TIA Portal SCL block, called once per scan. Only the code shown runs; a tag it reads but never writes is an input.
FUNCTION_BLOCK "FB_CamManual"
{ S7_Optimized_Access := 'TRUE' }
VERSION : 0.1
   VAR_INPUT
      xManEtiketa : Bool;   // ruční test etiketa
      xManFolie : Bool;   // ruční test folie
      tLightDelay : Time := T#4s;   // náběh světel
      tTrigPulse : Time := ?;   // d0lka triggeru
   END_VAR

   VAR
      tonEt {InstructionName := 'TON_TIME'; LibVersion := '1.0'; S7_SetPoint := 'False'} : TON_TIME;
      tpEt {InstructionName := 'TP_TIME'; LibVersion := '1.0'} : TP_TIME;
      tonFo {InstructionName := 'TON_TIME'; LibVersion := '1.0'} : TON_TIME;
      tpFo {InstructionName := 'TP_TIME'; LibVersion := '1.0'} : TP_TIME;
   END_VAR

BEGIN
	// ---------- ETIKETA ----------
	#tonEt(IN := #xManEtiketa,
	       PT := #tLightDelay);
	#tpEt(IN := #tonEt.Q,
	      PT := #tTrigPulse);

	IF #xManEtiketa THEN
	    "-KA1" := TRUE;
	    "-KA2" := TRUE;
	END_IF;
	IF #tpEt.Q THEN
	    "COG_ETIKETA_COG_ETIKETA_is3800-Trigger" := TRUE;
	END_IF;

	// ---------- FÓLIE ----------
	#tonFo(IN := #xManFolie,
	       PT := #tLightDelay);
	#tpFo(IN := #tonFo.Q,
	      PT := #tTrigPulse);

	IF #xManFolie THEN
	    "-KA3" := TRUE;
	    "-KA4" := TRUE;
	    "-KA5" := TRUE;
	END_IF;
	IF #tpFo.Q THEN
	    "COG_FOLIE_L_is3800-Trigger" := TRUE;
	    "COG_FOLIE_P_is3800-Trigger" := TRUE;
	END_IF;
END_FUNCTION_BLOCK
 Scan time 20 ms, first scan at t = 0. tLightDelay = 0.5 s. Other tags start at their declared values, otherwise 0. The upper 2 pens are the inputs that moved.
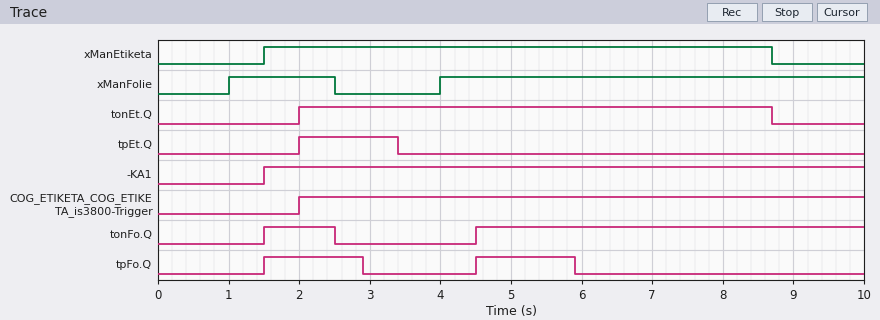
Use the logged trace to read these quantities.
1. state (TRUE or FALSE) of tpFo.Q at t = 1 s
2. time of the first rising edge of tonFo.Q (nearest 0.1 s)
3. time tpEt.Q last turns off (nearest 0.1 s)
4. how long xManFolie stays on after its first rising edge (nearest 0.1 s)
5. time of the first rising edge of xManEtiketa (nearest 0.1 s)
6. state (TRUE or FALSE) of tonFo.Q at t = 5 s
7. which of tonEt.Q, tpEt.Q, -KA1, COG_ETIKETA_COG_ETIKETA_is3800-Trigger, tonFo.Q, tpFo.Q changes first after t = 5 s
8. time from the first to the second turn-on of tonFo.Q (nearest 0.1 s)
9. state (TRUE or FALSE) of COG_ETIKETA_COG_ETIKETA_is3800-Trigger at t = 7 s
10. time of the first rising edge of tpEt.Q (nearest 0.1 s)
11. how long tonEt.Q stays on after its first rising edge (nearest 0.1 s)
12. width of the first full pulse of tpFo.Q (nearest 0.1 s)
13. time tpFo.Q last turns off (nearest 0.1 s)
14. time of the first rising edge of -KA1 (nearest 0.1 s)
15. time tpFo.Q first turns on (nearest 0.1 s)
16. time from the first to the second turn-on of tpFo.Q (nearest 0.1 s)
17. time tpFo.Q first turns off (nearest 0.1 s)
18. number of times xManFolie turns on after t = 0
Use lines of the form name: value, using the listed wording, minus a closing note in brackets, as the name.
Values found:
state (TRUE or FALSE) of tpFo.Q at t = 1 s: FALSE
time of the first rising edge of tonFo.Q: 1.5 s
time tpEt.Q last turns off: 3.4 s
how long xManFolie stays on after its first rising edge: 1.5 s
time of the first rising edge of xManEtiketa: 1.5 s
state (TRUE or FALSE) of tonFo.Q at t = 5 s: TRUE
which of tonEt.Q, tpEt.Q, -KA1, COG_ETIKETA_COG_ETIKETA_is3800-Trigger, tonFo.Q, tpFo.Q changes first after t = 5 s: tpFo.Q
time from the first to the second turn-on of tonFo.Q: 3.0 s
state (TRUE or FALSE) of COG_ETIKETA_COG_ETIKETA_is3800-Trigger at t = 7 s: TRUE
time of the first rising edge of tpEt.Q: 2.0 s
how long tonEt.Q stays on after its first rising edge: 6.7 s
width of the first full pulse of tpFo.Q: 1.4 s
time tpFo.Q last turns off: 5.9 s
time of the first rising edge of -KA1: 1.5 s
time tpFo.Q first turns on: 1.5 s
time from the first to the second turn-on of tpFo.Q: 3.0 s
time tpFo.Q first turns off: 2.9 s
number of times xManFolie turns on after t = 0: 2
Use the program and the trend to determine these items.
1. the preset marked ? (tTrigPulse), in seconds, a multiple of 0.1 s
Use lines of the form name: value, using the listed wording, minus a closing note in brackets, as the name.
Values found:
the preset marked ? (tTrigPulse), in seconds, a multiple of 0.1 s: 1.4 s
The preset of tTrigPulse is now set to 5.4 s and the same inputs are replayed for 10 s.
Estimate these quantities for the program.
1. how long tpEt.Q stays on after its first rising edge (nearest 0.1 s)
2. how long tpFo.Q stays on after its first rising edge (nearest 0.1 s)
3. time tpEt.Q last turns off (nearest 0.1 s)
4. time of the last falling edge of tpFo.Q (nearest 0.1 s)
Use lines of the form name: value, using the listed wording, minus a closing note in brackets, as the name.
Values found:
how long tpEt.Q stays on after its first rising edge: 5.4 s
how long tpFo.Q stays on after its first rising edge: 5.4 s
time tpEt.Q last turns off: 7.4 s
time of the last falling edge of tpFo.Q: 6.9 s
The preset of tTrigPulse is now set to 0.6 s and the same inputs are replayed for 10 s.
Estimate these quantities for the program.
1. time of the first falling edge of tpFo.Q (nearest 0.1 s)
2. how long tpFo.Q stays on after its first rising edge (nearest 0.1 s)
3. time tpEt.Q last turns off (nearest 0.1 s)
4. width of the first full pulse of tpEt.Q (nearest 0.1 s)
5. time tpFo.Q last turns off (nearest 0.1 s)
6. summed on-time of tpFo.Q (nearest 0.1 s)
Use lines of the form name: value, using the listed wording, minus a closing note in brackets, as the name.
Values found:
time of the first falling edge of tpFo.Q: 2.1 s
how long tpFo.Q stays on after its first rising edge: 0.6 s
time tpEt.Q last turns off: 2.6 s
width of the first full pulse of tpEt.Q: 0.6 s
time tpFo.Q last turns off: 5.1 s
summed on-time of tpFo.Q: 1.2 s
